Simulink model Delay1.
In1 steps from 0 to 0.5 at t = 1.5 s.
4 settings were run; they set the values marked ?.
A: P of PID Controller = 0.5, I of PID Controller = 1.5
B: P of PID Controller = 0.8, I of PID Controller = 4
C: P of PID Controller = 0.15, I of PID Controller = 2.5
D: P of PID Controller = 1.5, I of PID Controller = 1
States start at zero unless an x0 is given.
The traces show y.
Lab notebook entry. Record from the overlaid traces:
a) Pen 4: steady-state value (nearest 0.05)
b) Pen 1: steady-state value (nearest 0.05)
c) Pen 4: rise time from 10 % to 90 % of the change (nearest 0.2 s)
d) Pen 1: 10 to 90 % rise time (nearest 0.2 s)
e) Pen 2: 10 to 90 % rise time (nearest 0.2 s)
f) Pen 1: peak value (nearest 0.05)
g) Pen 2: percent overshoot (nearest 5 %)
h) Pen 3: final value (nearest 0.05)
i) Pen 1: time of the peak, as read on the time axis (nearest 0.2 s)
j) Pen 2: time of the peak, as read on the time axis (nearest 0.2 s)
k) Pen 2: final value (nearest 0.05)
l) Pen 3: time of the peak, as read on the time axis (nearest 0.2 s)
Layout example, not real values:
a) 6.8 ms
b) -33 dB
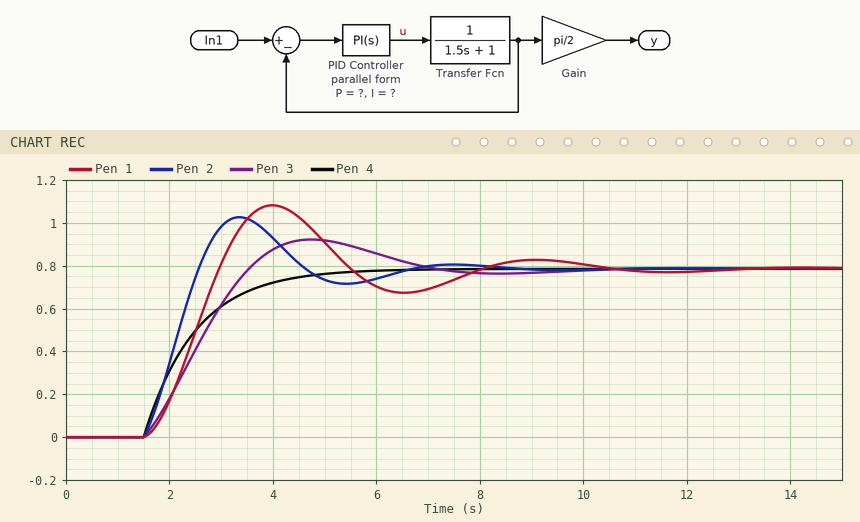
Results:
a) 0.80
b) 0.80
c) 2.2 s
d) 1.0 s
e) 0.8 s
f) 1.10
g) 30 %
h) 0.80
i) 4.0 s
j) 3.4 s
k) 0.80
l) 4.8 s
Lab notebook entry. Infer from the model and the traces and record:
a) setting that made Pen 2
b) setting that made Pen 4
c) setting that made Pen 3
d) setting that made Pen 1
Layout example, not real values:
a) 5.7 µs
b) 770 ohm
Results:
a) B
b) D
c) A
d) C
